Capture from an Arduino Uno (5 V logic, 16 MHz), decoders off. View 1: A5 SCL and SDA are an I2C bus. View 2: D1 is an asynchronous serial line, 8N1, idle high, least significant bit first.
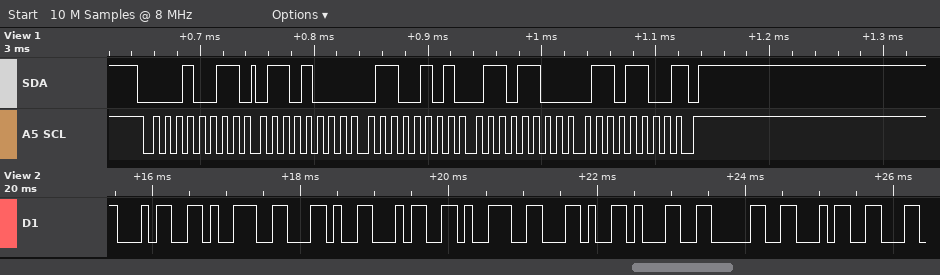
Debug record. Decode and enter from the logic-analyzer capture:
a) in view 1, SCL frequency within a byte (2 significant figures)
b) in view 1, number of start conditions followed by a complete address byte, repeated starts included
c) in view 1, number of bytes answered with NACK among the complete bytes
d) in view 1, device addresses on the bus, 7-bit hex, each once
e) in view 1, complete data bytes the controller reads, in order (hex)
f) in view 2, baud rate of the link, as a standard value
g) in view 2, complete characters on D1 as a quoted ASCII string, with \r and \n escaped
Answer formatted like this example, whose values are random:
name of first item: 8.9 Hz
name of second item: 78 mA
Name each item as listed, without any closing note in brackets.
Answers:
in view 1, SCL frequency within a byte: 100 kHz
in view 1, number of start conditions followed by a complete address byte, repeated starts included: 1
in view 1, number of bytes answered with NACK among the complete bytes: 1
in view 1, device addresses on the bus, 7-bit hex, each once: 0x09
in view 1, complete data bytes the controller reads, in order: 68 65 6C 6C
in view 2, baud rate of the link, as a standard value: 9600 baud
in view 2, complete characters on D1 as a quoted ASCII string, with \r and \n escaped: "49,49,104"
